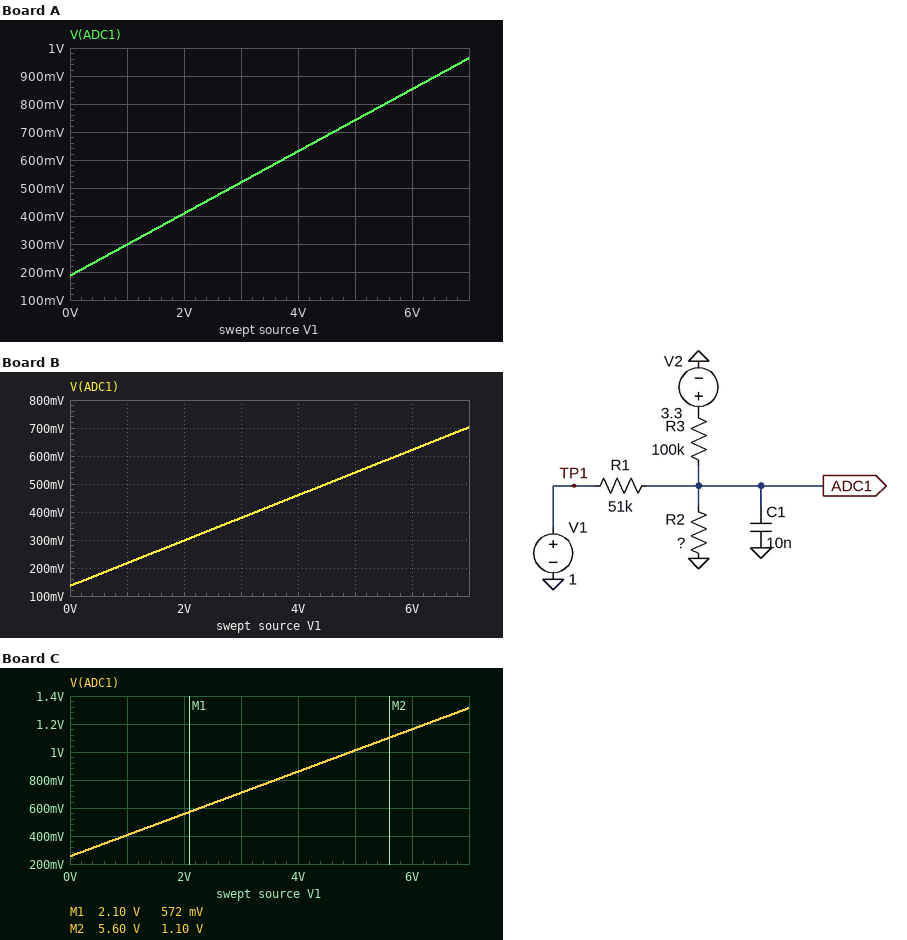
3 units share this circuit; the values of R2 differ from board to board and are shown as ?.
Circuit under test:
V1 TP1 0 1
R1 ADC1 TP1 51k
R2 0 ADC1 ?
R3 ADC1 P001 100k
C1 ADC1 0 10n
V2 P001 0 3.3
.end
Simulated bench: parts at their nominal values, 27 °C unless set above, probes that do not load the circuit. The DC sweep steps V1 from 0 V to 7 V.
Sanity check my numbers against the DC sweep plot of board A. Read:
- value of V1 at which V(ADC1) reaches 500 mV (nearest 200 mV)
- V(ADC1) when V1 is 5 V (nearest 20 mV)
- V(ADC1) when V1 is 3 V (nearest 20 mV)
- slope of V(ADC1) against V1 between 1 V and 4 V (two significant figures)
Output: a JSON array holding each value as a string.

["2.8 V", "740 mV", "520 mV", "0.11 V/V"]
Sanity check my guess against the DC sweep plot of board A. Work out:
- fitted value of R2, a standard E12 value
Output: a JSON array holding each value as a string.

["6.8 kΩ"]
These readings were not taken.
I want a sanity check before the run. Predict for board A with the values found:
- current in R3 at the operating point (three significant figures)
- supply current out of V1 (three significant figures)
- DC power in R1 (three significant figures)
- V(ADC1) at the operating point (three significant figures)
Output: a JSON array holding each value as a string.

["30.0 µA", "13.8 µA", "9.67 µW", "298 mV"]
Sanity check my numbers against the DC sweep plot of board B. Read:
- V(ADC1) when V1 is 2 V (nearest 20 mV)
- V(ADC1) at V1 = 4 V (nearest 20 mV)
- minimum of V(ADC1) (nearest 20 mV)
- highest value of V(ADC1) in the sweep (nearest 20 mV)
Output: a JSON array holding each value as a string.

["300 mV", "460 mV", "140 mV", "700 mV"]
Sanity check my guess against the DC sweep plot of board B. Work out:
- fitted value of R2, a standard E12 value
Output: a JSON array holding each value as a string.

["4.7 kΩ"]
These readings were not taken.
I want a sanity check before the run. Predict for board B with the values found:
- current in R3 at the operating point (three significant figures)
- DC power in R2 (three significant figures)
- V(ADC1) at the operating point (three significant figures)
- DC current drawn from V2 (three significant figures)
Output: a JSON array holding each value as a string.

["30.8 µA", "10.0 µW", "217 mV", "30.8 µA"]
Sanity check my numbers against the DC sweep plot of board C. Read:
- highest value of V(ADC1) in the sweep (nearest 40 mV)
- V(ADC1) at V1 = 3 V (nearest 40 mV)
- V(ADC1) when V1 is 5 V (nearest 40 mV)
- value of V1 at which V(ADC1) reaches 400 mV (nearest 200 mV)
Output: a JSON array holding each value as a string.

["1.32 V", "720 mV", "1.00 V", "1.0 V"]
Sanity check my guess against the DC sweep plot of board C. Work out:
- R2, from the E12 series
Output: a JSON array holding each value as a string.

["10 kΩ"]
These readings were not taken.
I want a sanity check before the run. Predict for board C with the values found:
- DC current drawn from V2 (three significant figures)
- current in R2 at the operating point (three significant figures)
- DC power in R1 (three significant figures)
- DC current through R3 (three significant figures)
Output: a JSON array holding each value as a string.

["28.9 µA", "40.6 µA", "6.92 µW", "28.9 µA"]
